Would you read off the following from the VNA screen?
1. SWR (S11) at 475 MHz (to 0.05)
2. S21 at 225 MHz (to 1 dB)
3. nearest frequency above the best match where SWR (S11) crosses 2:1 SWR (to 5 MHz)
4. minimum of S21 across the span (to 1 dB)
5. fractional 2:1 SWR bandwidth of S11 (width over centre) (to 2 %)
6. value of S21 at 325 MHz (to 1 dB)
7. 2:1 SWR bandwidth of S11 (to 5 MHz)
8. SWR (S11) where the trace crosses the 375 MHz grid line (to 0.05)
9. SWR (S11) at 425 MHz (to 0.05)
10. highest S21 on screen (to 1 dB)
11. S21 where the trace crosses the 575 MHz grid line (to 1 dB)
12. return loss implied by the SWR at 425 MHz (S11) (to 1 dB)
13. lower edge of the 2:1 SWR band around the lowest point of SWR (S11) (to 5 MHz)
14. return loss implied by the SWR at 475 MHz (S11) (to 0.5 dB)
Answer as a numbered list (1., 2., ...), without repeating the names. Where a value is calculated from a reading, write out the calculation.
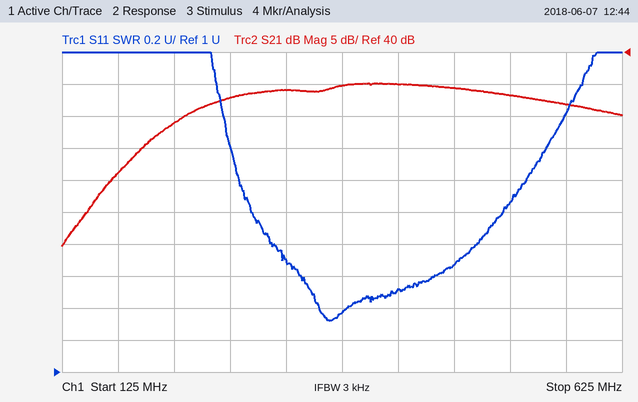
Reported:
1. 1.65
2. 29 dB
3. 520 MHz
4. 10 dB
5. 225 MHz / 407.5 MHz ≈ 55.2 %, so 56 % to the nearest 2 %
6. 34 dB
7. 520 MHz − 295 MHz = 225 MHz
8. 1.35
9. 1.50
10. 35 dB
11. 32 dB
12. −20 log10((1.5 − 1)/(1.5 + 1)) ≈ 14 dB
13. 295 MHz
14. −20 log10((1.65 − 1)/(1.65 + 1)) ≈ 12.2 dB, so 12.0 dB to the nearest 0.5 dB
